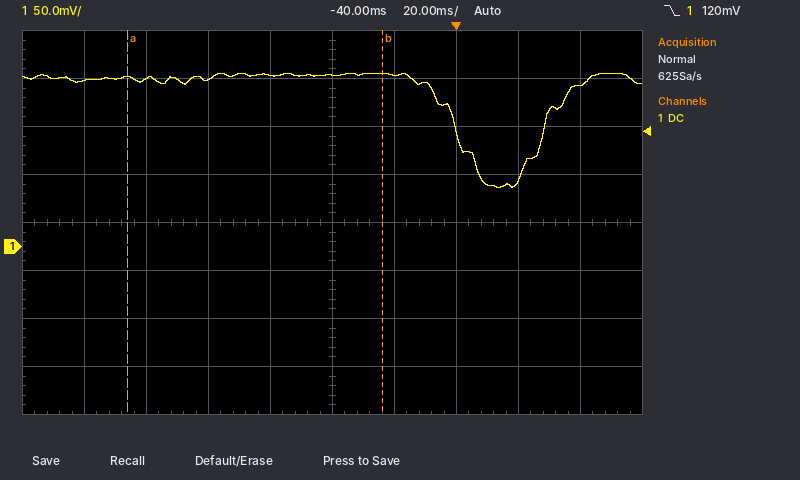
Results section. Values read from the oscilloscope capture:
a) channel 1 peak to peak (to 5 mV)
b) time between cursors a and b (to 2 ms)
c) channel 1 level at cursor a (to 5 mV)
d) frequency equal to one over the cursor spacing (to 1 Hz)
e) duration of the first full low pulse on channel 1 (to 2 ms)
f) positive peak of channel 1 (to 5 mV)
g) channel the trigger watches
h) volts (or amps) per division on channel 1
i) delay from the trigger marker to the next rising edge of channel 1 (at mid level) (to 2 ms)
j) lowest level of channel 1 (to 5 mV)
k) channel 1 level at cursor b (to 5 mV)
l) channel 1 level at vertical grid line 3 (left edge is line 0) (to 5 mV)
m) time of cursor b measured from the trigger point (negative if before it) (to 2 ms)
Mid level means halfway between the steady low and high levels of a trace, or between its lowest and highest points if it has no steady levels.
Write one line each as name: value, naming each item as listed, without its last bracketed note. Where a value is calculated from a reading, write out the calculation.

channel 1 peak to peak: 180 mV − (60 mV) = 120 mV
time between cursors a and b: 82 ms
channel 1 level at cursor a: 175 mV
frequency equal to one over the cursor spacing: 1 / 82 ms ≈ 12 Hz
duration of the first full low pulse on channel 1: 28 ms
positive peak of channel 1: 180 mV
channel the trigger watches: channel 1
volts (or amps) per division on channel 1: 50 mV
delay from the trigger marker to the next rising edge of channel 1 (at mid level): 28 ms
lowest level of channel 1: 60 mV
channel 1 level at cursor b: 180 mV
channel 1 level at vertical grid line 3 (left edge is line 0): 175 mV
time of cursor b measured from the trigger point (negative if before it): -24 ms
